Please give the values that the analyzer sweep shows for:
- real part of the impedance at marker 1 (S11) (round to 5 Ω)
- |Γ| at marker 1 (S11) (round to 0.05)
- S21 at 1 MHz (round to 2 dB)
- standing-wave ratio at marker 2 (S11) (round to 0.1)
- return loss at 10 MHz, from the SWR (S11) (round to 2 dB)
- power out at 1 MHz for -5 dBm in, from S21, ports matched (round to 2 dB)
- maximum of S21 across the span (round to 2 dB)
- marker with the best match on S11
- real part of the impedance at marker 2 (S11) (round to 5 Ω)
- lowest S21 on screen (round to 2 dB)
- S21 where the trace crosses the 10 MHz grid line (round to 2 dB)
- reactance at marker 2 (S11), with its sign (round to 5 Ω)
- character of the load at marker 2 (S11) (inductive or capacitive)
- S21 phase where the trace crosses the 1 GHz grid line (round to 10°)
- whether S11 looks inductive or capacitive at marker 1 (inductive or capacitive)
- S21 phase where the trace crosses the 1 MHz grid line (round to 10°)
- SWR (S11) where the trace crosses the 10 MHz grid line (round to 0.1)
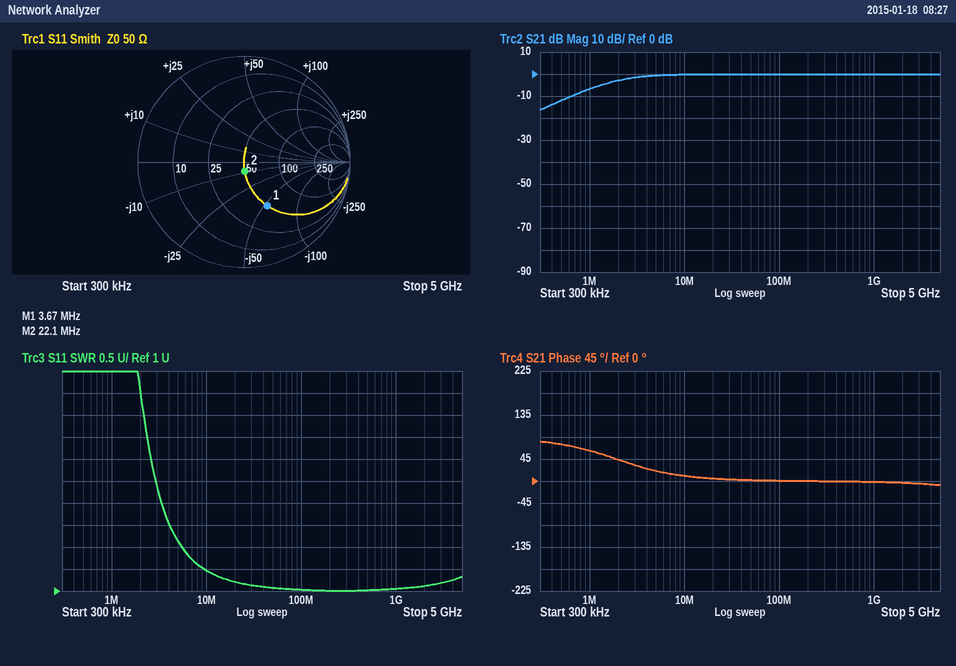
50 Ω
0.45
-6 dB
1.2
14 dB
-12 dBm
0 dB
marker 2
50 Ω
-16 dB
0 dB
-10 Ω
capacitive
0°
capacitive
60°
1.5
